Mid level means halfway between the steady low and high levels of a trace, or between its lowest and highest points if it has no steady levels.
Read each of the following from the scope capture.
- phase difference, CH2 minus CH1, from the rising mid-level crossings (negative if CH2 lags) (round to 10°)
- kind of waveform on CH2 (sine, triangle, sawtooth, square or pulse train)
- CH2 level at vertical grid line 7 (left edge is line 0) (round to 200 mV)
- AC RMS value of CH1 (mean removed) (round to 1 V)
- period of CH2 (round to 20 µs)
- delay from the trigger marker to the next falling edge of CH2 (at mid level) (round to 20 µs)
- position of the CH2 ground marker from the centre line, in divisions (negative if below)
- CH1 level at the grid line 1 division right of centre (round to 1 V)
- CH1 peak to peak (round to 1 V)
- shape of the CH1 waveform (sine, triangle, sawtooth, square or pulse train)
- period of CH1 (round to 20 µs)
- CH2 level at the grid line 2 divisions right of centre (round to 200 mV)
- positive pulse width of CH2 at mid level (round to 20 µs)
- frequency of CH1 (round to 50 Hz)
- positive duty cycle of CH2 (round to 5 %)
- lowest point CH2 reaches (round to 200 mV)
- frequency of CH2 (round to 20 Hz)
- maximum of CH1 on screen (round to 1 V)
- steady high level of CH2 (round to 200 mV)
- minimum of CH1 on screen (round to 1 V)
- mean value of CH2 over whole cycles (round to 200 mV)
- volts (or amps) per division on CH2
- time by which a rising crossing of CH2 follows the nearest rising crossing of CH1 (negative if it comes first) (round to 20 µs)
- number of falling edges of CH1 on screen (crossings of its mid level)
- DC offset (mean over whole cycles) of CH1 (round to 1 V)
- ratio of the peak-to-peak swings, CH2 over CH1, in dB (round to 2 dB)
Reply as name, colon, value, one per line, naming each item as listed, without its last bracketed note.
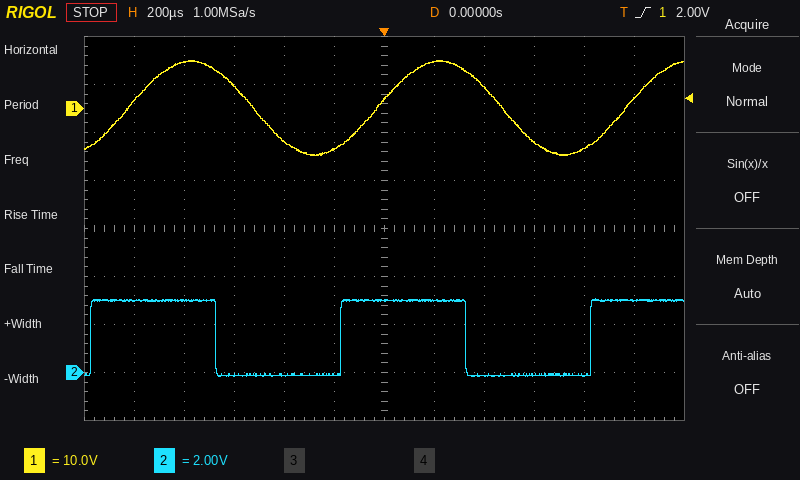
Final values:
phase difference, CH2 minus CH1, from the rising mid-level crossings (negative if CH2 lags): +50°
kind of waveform on CH2: square
CH2 level at vertical grid line 7 (left edge is line 0): 3.0 V
AC RMS value of CH1 (mean removed): 7 V
period of CH2: 1.00 ms
delay from the trigger marker to the next falling edge of CH2 (at mid level): 320 µs
position of the CH2 ground marker from the centre line, in divisions: -3.0 div
CH1 level at the grid line 1 division right of centre: 10 V
CH1 peak to peak: 20 V
shape of the CH1 waveform: sine
period of CH1: 1.00 ms
CH2 level at the grid line 2 divisions right of centre: -200 mV
positive pulse width of CH2 at mid level: 500 µs
frequency of CH1: 1.00 kHz
positive duty cycle of CH2: 50 %
lowest point CH2 reaches: -200 mV
frequency of CH2: 1.00 kHz
maximum of CH1 on screen: 10 V
steady high level of CH2: 3.0 V
minimum of CH1 on screen: -10 V
mean value of CH2 over whole cycles: 1.4 V
volts (or amps) per division on CH2: 2 V
time by which a rising crossing of CH2 follows the nearest rising crossing of CH1 (negative if it comes first): -140 µs
number of falling edges of CH1 on screen: 2
DC offset (mean over whole cycles) of CH1: 0 V
ratio of the peak-to-peak swings, CH2 over CH1, in dB: -16 dB
